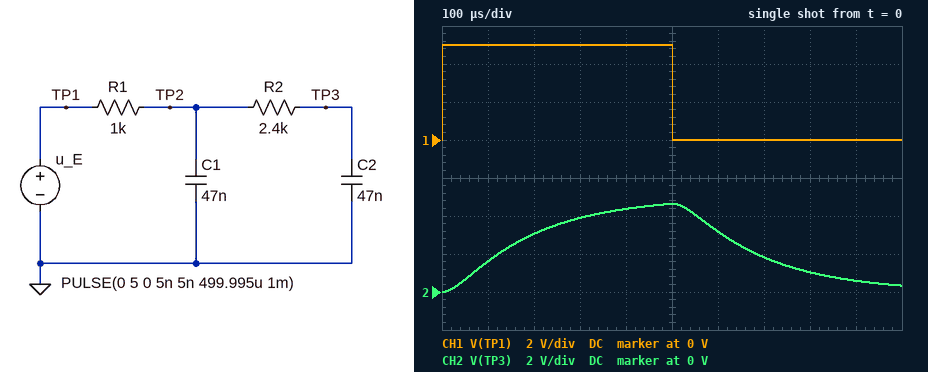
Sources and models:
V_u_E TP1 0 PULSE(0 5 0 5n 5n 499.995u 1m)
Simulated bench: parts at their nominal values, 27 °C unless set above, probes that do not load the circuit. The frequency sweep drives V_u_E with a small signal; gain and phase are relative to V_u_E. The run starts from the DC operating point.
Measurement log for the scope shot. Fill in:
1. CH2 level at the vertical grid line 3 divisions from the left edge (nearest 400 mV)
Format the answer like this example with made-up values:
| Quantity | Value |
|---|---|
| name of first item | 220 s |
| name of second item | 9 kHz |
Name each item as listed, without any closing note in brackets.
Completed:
| Quantity | Value |
|---|---|
| CH2 level at the vertical grid line 3 divisions from the left edge | 4.0 V |
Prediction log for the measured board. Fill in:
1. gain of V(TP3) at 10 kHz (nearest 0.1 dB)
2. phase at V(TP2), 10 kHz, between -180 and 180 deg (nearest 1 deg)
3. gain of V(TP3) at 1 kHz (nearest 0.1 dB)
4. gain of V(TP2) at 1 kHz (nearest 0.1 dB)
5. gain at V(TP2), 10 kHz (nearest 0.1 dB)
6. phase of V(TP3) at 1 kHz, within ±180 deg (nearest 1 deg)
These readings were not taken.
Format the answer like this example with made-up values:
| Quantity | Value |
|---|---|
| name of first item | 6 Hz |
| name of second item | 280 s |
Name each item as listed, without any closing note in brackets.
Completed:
| Quantity | Value |
|---|---|
| gain of V(TP3) at 10 kHz | -27.5 dB |
| phase at V(TP2), 10 kHz, between -180 and 180 deg | -65 deg |
| gain of V(TP3) at 1 kHz | -3.6 dB |
| gain of V(TP2) at 1 kHz | -1.9 dB |
| gain at V(TP2), 10 kHz | -10.4 dB |
| phase of V(TP3) at 1 kHz, within ±180 deg | -59 deg |
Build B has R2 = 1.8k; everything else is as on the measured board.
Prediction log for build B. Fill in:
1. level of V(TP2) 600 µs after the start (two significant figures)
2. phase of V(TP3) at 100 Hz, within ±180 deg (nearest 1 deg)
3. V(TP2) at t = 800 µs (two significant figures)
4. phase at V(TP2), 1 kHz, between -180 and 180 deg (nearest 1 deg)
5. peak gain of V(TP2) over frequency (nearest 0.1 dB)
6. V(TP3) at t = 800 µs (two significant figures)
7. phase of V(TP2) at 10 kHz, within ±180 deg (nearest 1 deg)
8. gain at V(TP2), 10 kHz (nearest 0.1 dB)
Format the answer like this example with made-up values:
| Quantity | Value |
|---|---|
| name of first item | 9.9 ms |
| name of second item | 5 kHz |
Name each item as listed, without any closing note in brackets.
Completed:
| Quantity | Value |
|---|---|
| level of V(TP2) 600 µs after the start | 1.4 V |
| phase of V(TP3) at 100 Hz, within ±180 deg | -6 deg |
| V(TP2) at t = 800 µs | 360 mV |
| phase at V(TP2), 1 kHz, between -180 and 180 deg | -25 deg |
| peak gain of V(TP2) over frequency | 0 dB |
| V(TP3) at t = 800 µs | 810 mV |
| phase of V(TP2) at 10 kHz, within ±180 deg | -63 deg |
| gain at V(TP2), 10 kHz | -10.7 dB |
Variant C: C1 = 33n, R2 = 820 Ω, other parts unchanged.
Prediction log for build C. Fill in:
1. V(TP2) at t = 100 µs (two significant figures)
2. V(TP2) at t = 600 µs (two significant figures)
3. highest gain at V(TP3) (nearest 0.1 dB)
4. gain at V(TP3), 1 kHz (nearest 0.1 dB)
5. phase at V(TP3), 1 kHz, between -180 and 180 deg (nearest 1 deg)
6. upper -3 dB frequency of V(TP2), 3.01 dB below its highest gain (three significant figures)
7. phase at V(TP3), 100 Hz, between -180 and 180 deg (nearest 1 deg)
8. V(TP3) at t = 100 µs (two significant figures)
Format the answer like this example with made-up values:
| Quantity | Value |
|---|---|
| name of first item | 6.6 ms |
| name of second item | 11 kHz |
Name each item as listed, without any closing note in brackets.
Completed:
| Quantity | Value |
|---|---|
| V(TP2) at t = 100 µs | 3.6 V |
| V(TP2) at t = 600 µs | 1.4 V |
| highest gain at V(TP3) | 0 dB |
| gain at V(TP3), 1 kHz | -1.6 dB |
| phase at V(TP3), 1 kHz, between -180 and 180 deg | -38 deg |
| upper -3 dB frequency of V(TP2), 3.01 dB below its highest gain | 1.70 kHz |
| phase at V(TP3), 100 Hz, between -180 and 180 deg | -4 deg |
| V(TP3) at t = 100 µs | 2.8 V |
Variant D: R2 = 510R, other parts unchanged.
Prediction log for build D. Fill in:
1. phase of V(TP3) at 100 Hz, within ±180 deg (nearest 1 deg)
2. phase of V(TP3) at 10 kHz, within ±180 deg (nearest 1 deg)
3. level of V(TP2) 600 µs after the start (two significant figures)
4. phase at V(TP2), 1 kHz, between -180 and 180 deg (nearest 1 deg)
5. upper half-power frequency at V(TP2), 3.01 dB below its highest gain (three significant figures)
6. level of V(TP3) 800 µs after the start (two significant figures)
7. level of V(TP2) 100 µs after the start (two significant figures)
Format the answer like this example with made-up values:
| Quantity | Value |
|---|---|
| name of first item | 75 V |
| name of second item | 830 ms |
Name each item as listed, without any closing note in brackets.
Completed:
| Quantity | Value |
|---|---|
| phase of V(TP3) at 100 Hz, within ±180 deg | -4 deg |
| phase of V(TP3) at 10 kHz, within ±180 deg | -115 deg |
| level of V(TP2) 600 µs after the start | 1.7 V |
| phase at V(TP2), 1 kHz, between -180 and 180 deg | -29 deg |
| upper half-power frequency at V(TP2), 3.01 dB below its highest gain | 1.54 kHz |
| level of V(TP3) 800 µs after the start | 340 mV |
| level of V(TP2) 100 µs after the start | 3.3 V |
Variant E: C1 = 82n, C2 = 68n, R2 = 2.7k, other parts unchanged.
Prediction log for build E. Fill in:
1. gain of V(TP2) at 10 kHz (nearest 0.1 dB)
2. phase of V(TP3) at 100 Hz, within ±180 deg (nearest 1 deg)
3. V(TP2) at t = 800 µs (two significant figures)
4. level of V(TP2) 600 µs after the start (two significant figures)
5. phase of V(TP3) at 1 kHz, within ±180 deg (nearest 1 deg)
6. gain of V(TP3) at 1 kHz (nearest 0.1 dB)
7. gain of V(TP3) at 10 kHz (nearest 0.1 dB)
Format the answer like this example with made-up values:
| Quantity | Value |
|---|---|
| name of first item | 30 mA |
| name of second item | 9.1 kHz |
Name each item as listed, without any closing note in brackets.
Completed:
| Quantity | Value |
|---|---|
| gain of V(TP2) at 10 kHz | -14.6 dB |
| phase of V(TP3) at 100 Hz, within ±180 deg | -12 deg |
| V(TP2) at t = 800 µs | 620 mV |
| level of V(TP2) 600 µs after the start | 1.7 V |
| phase of V(TP3) at 1 kHz, within ±180 deg | -79 deg |
| gain of V(TP3) at 1 kHz | -6.6 dB |
| gain of V(TP3) at 10 kHz | -35.9 dB |
